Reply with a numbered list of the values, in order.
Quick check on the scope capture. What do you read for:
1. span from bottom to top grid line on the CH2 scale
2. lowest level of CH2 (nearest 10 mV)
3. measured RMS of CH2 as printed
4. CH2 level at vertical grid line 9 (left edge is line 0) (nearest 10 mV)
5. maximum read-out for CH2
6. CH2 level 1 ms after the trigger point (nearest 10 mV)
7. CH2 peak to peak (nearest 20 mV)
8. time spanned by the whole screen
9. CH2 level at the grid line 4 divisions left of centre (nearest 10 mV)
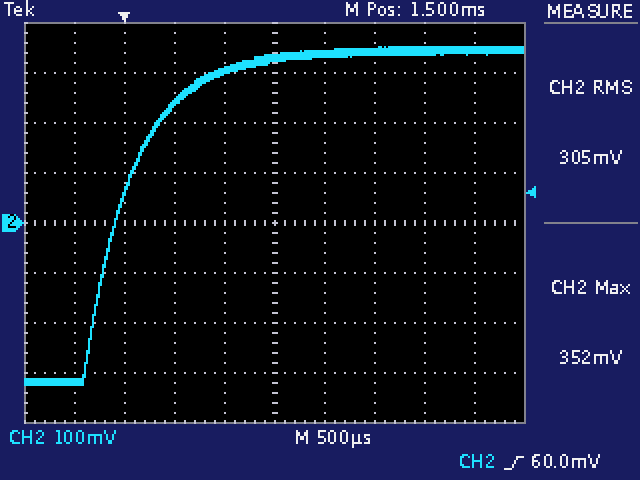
1. 800 mV
2. -320 mV
3. 305 mV
4. 350 mV
5. 352 mV
6. 300 mV
7. 680 mV
8. 5 ms
9. -320 mV
